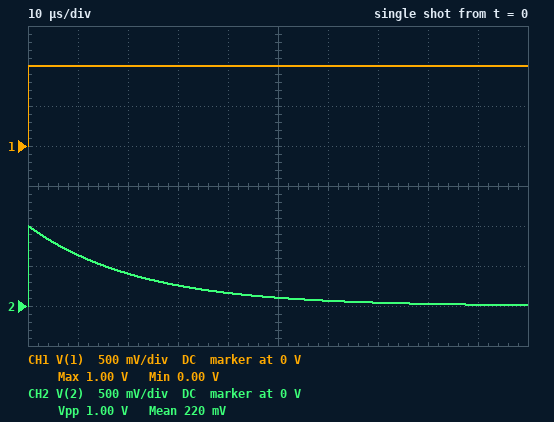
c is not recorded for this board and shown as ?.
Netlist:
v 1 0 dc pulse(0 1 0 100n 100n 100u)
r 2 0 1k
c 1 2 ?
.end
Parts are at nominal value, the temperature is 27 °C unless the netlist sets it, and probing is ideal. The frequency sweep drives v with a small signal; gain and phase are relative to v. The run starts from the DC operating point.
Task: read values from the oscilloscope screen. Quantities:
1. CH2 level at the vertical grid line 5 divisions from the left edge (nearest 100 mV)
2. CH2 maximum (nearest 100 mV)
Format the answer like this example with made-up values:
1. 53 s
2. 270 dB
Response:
1. 100 mV
2. 1.0 V
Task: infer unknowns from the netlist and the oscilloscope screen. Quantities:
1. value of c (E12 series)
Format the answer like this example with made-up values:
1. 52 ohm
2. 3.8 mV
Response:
1. 22 nF
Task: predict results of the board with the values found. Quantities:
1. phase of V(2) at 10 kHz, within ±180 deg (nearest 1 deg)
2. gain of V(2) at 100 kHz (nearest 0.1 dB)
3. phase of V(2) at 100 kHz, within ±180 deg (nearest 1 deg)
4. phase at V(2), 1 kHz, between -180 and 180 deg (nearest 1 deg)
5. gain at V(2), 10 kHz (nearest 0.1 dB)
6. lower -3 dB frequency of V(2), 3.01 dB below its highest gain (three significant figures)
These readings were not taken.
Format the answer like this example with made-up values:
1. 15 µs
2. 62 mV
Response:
1. 36 deg
2. 0 dB
3. 4 deg
4. 82 deg
5. -1.8 dB
6. 7.23 kHz
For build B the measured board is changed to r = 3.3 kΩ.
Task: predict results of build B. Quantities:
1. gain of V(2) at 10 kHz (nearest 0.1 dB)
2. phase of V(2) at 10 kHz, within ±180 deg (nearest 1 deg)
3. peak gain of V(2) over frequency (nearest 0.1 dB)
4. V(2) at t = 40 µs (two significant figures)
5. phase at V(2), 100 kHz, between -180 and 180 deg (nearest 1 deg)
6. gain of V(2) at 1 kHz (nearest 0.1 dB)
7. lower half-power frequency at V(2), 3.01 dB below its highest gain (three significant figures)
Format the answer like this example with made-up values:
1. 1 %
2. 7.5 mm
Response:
1. -0.2 dB
2. 12 deg
3. 0 dB
4. 580 mV
5. 1 deg
6. -7.6 dB
7. 2.19 kHz
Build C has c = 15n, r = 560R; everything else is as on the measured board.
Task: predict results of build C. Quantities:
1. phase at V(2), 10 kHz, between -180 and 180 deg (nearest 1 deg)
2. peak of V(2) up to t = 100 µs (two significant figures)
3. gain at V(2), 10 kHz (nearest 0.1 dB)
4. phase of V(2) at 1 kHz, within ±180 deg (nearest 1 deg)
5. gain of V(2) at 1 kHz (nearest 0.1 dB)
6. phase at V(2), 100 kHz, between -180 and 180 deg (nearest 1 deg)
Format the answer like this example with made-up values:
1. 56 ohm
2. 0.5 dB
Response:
1. 62 deg
2. 990 mV
3. -6.6 dB
4. 87 deg
5. -25.6 dB
6. 11 deg
